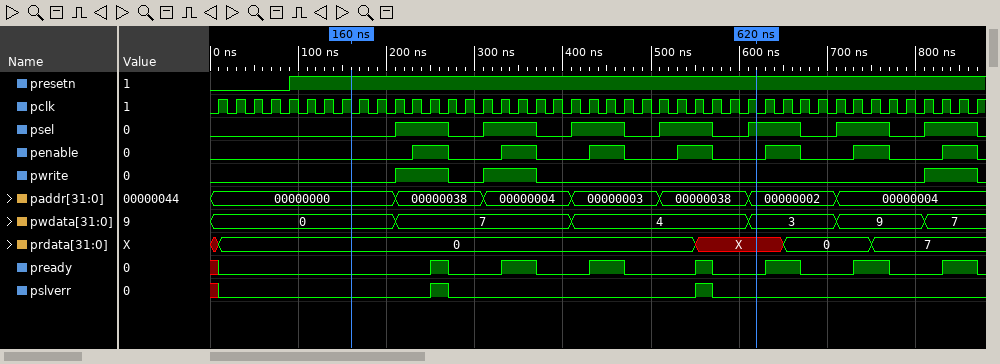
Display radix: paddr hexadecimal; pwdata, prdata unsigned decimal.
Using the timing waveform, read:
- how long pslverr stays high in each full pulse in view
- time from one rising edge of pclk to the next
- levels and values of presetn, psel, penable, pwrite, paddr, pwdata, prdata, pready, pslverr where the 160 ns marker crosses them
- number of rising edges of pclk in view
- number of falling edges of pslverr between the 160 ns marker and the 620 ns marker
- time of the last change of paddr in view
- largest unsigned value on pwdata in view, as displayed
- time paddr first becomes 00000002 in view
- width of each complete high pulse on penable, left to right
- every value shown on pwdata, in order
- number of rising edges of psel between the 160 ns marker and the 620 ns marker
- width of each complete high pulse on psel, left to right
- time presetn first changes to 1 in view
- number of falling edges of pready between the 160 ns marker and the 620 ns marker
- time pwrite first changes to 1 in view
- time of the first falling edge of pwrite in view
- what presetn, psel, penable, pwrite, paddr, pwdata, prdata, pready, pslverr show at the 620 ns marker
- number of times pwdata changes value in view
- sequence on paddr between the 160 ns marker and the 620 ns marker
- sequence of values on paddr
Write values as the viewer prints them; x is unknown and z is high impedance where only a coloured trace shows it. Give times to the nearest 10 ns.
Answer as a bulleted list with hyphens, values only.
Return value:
- 20 ns, 20 ns
- 20 ns
- presetn=1, psel=0, penable=0, pwrite=0, paddr=00000000, pwdata=0, prdata=0, pready=0, pslverr=0
- 44
- 2
- 710 ns
- 9
- 610 ns
- 40 ns, 40 ns, 40 ns, 40 ns, 40 ns, 40 ns, 40 ns
- 0, 7, 4, 3, 9, 7
- 5
- 60 ns, 60 ns, 60 ns, 60 ns, 60 ns, 60 ns, 60 ns
- 90 ns
- 4
- 210 ns
- 270 ns
- presetn=1, psel=1, penable=0, pwrite=0, paddr=00000002, pwdata=3, prdata=X, pready=0, pslverr=0
- 5
- 00000000, 00000038, 00000004, 00000003, 00000038, 00000002
- 00000000, 00000038, 00000004, 00000003, 00000038, 00000002, 00000004
